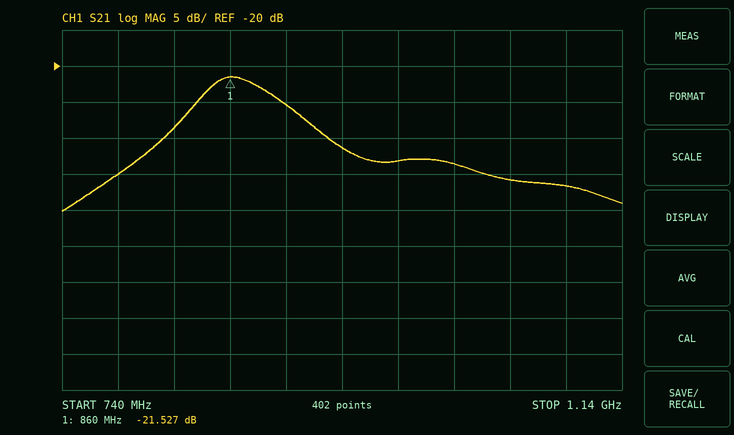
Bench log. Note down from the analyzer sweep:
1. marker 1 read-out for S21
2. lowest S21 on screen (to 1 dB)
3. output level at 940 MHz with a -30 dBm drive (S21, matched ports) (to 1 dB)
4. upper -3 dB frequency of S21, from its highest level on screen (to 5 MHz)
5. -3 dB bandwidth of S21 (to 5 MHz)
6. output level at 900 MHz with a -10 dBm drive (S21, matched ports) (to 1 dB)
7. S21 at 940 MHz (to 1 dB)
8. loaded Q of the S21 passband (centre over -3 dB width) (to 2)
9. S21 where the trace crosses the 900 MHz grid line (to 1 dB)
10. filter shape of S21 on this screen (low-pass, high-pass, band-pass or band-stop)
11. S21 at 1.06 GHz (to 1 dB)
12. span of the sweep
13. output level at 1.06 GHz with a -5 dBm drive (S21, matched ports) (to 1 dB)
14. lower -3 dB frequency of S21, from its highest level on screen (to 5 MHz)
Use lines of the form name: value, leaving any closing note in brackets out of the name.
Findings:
marker 1 read-out for S21: -21.527 dB
lowest S21 on screen: -40 dB
output level at 940 MHz with a -30 dBm drive (S21, matched ports): -61 dBm
upper -3 dB frequency of S21, from its highest level on screen: 895 MHz
-3 dB bandwidth of S21: 55 MHz
output level at 900 MHz with a -10 dBm drive (S21, matched ports): -35 dBm
S21 at 940 MHz: -31 dB
loaded Q of the S21 passband (centre over -3 dB width): 16
S21 where the trace crosses the 900 MHz grid line: -25 dB
filter shape of S21 on this screen: band-pass
S21 at 1.06 GHz: -36 dB
span of the sweep: 400 MHz
output level at 1.06 GHz with a -5 dBm drive (S21, matched ports): -41 dBm
lower -3 dB frequency of S21, from its highest level on screen: 840 MHz
